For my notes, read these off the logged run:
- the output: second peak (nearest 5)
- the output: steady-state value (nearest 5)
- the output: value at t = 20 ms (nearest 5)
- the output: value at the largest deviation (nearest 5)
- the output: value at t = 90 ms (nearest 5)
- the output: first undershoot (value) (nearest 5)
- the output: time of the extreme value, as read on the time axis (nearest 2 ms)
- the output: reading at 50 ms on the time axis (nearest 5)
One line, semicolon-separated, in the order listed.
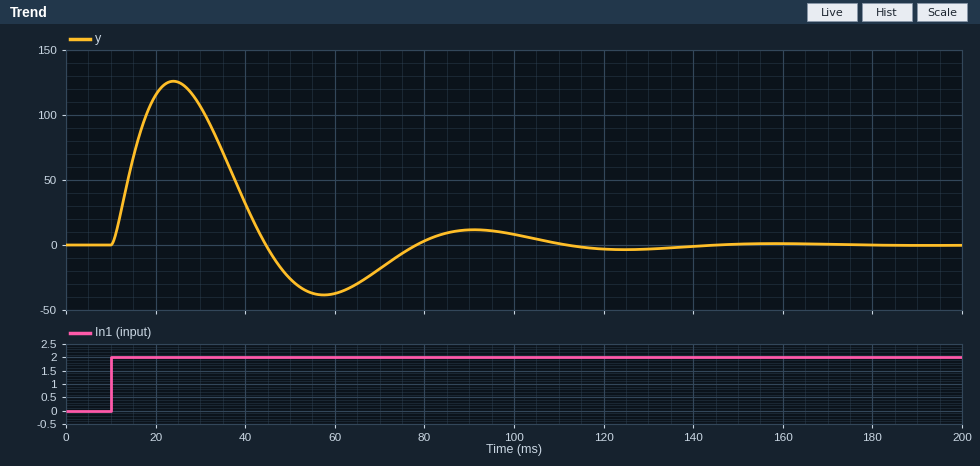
10; 0; 115; 125; 10; -40; 24 ms; -25
